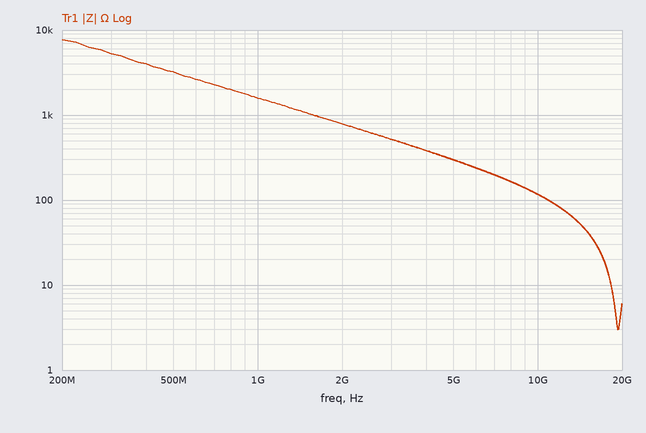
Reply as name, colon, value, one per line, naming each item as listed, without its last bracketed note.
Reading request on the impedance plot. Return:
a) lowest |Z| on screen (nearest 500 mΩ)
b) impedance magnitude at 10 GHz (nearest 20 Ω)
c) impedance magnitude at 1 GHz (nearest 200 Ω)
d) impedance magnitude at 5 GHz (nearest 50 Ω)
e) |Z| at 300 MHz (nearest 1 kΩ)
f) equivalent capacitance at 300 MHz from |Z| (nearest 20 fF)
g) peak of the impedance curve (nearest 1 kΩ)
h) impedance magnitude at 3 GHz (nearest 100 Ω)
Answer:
lowest |Z| on screen: 3.0 Ω
impedance magnitude at 10 GHz: 120 Ω
impedance magnitude at 1 GHz: 1.6 kΩ
impedance magnitude at 5 GHz: 300 Ω
|Z| at 300 MHz: 5 kΩ
equivalent capacitance at 300 MHz from |Z|: 100 fF
peak of the impedance curve: 8 kΩ
impedance magnitude at 3 GHz: 500 Ω
